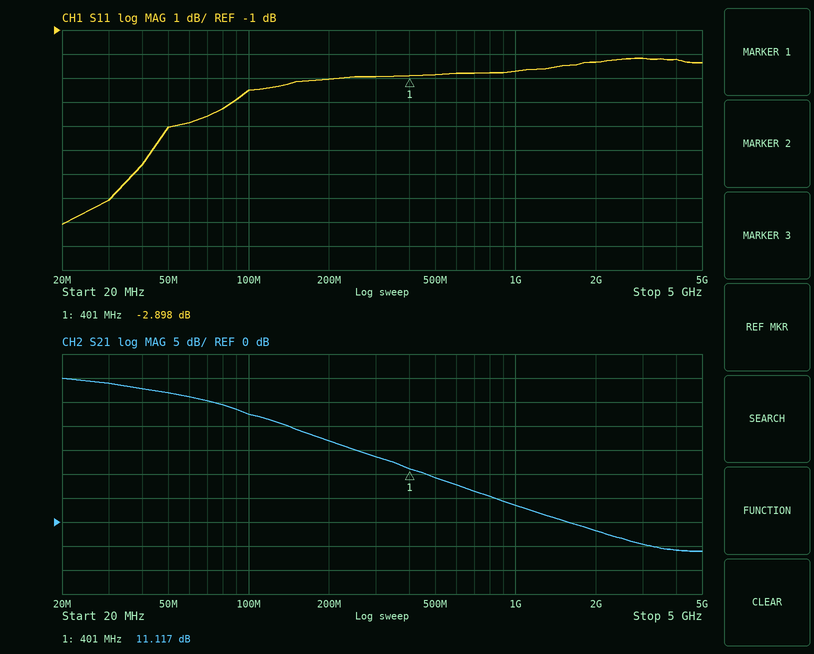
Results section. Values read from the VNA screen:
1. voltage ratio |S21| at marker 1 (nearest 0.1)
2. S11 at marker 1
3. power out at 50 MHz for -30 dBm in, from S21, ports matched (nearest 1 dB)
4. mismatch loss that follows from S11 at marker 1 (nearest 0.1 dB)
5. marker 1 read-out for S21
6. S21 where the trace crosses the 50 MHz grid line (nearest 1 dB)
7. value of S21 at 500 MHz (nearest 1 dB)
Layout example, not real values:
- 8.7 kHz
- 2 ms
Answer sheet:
- 3.6
- -2.898 dB
- -3 dBm
- 3.1 dB
- 11.117 dB
- 27 dB
- 9 dB
